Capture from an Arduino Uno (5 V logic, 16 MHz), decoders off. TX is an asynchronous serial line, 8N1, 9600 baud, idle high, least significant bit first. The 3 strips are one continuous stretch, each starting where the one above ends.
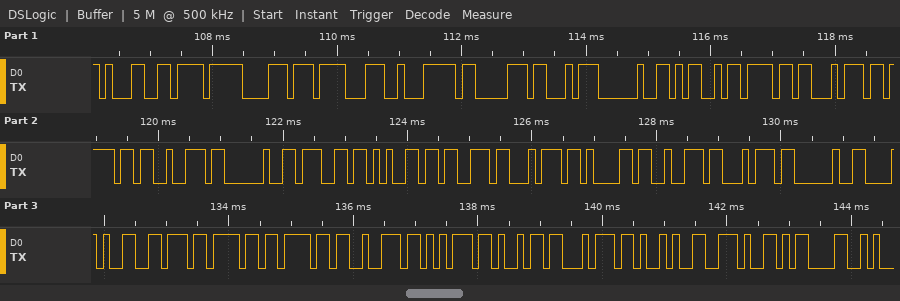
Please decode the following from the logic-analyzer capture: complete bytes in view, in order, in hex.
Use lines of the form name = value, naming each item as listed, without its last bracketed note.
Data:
complete bytes in view, in order, in hex = 31 EF B8 8F E2 83 A3 20 4D 6F 74 6F 72 20 67 65 73 74 61 72 74 20 28 76 6F 6F 72 75 69 74 29 2E 0D
